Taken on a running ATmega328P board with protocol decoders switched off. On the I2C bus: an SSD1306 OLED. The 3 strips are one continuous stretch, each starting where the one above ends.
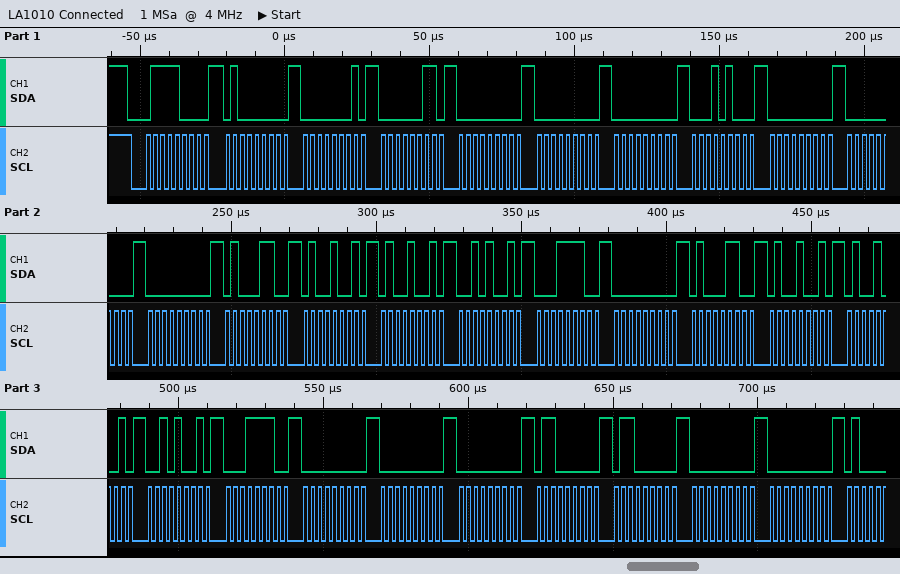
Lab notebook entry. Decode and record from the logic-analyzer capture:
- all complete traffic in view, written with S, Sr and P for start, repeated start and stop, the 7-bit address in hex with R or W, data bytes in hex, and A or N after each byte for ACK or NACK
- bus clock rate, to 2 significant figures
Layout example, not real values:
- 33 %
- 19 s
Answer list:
- S 3CW A 40 A 01 A 03 A 00 A 00 A 00 A 14 A 00 A 00 A 00 A 46 A 49 A 49 A 29 A 1E A 00 A 46 A 49 A 49 A 29 A 1E A 00 A 00 A 00 A 60 A 60 A 00 A 00 A
- 400 kHz
